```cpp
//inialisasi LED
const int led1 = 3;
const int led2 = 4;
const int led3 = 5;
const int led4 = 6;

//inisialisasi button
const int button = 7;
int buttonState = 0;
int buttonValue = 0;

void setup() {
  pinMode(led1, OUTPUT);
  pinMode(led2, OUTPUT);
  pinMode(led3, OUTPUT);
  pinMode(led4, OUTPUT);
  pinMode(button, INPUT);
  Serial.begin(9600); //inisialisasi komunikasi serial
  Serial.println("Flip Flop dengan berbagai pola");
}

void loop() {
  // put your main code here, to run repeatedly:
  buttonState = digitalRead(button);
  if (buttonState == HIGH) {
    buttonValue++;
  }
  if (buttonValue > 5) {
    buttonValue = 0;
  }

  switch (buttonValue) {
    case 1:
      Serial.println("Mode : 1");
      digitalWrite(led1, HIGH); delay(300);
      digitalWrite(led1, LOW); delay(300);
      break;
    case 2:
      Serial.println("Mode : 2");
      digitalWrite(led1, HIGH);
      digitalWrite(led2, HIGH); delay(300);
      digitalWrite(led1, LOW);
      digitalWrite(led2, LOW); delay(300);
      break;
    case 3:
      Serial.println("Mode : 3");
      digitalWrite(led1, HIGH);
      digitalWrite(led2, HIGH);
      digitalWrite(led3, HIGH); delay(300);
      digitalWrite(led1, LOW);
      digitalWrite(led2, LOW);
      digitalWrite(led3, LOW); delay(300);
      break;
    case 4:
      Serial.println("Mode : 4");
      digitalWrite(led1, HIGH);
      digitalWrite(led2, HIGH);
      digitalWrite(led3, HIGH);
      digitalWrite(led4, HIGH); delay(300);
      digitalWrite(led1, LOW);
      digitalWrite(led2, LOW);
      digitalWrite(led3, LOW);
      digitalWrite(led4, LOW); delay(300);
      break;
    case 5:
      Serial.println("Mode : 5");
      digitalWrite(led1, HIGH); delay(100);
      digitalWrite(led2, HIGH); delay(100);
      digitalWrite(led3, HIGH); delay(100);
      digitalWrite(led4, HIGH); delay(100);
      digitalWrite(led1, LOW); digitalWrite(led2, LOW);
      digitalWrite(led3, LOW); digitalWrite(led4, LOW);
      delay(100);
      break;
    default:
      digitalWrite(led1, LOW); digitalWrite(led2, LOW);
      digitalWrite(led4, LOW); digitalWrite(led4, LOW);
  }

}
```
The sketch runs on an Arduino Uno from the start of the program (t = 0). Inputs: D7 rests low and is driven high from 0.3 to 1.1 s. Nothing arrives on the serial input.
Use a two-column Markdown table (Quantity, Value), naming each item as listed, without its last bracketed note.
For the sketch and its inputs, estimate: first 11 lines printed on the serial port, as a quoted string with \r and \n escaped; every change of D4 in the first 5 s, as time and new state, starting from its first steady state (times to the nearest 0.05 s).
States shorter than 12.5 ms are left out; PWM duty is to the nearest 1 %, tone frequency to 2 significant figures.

| Quantity | Value |
|---|---|
| first 11 lines printed on the serial port, as a quoted string with \r and \n escaped | "Flip Flop dengan berbagai pola\r\nMode : 1\r\nMode : 2\r\nMode : 2\r\nMode : 2\r\nMode : 2\r\nMode : 2\r\nMode : 2\r\nMode : 2\r\nMode : 2\r\nMode : 2\r\n" |
| every change of D4 in the first 5 s, as time and new state, starting from its first steady state | 0 s low; 0.9 s high; 1.2 s low; 1.5 s high; 1.8 s low; 2.1 s high; 2.4 s low; 2.7 s high; 3 s low; 3.3 s high; 3.6 s low; 3.9 s high; 4.2 s low; 4.5 s high; 4.8 s low |
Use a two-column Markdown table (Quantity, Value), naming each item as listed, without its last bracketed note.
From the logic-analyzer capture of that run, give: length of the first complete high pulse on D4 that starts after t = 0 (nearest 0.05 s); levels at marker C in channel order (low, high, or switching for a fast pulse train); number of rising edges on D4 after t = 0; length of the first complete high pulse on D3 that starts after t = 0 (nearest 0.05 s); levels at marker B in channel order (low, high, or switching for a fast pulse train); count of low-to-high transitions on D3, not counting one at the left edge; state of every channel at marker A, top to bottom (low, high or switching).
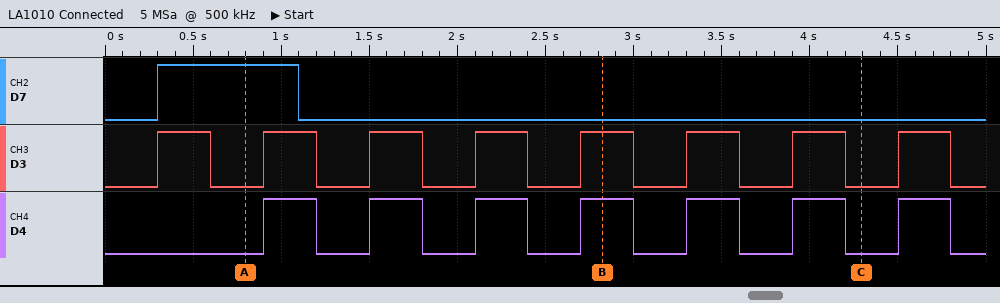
| Quantity | Value |
|---|---|
| length of the first complete high pulse on D4 that starts after t = 0 | 0.30 s |
| levels at marker C in channel order | D7 low, D3 low, D4 low |
| number of rising edges on D4 after t = 0 | 7 |
| length of the first complete high pulse on D3 that starts after t = 0 | 0.30 s |
| levels at marker B in channel order | D7 low, D3 high, D4 high |
| count of low-to-high transitions on D3, not counting one at the left edge | 8 |
| state of every channel at marker A, top to bottom | D7 high, D3 low, D4 low |
